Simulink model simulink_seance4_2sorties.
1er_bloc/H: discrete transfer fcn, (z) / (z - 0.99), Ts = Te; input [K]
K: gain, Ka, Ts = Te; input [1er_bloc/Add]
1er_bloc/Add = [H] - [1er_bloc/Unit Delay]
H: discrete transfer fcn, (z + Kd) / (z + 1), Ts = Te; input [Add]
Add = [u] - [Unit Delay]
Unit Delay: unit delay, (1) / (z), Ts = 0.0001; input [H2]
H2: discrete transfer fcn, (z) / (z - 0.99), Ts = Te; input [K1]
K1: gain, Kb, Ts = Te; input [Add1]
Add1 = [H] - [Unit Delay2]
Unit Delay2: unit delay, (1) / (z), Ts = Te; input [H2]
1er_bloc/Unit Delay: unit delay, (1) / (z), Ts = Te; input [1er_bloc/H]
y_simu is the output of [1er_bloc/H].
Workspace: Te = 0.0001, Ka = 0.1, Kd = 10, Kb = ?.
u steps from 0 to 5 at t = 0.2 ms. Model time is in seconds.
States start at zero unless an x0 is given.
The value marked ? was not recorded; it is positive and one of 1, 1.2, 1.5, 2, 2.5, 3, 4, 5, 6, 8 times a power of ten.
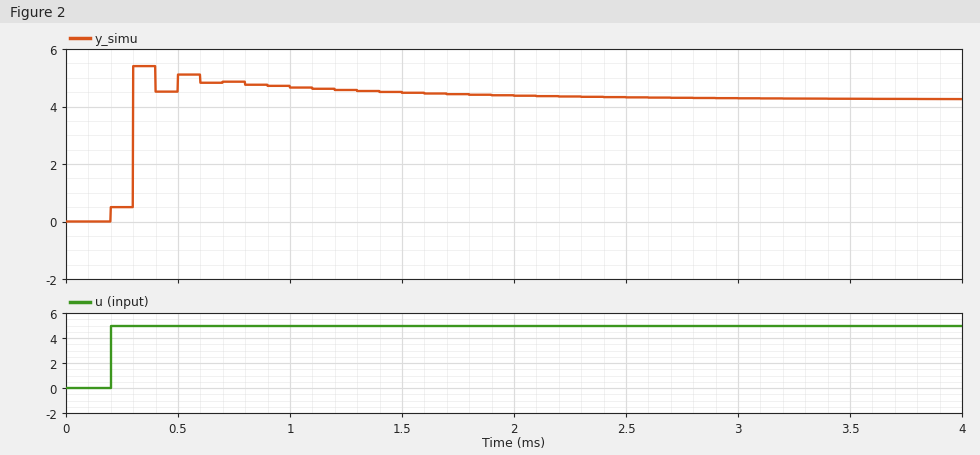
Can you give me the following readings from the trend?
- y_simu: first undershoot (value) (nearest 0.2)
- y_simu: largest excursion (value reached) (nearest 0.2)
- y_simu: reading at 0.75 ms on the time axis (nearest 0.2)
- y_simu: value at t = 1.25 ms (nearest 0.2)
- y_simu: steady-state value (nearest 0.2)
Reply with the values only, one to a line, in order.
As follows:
4.6
5.4
4.8
4.6
4.2
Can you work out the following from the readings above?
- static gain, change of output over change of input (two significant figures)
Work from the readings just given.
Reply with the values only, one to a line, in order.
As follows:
0.84
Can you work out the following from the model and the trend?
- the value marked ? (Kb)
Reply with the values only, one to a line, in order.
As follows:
0.08
